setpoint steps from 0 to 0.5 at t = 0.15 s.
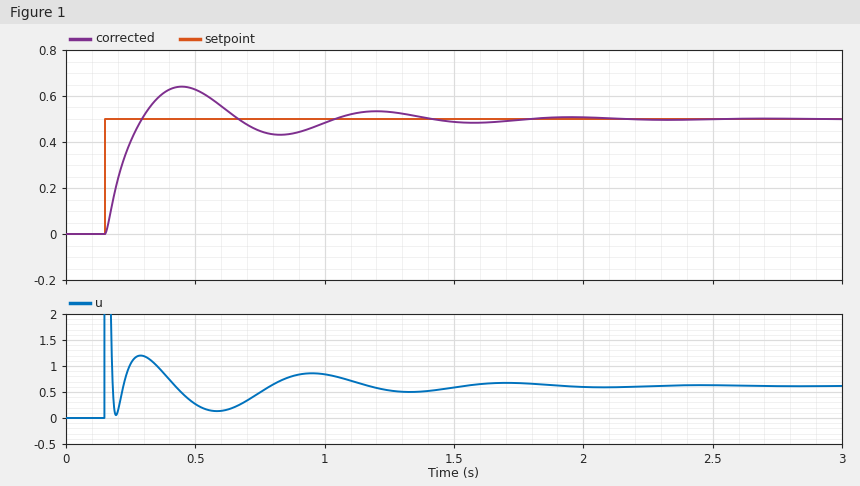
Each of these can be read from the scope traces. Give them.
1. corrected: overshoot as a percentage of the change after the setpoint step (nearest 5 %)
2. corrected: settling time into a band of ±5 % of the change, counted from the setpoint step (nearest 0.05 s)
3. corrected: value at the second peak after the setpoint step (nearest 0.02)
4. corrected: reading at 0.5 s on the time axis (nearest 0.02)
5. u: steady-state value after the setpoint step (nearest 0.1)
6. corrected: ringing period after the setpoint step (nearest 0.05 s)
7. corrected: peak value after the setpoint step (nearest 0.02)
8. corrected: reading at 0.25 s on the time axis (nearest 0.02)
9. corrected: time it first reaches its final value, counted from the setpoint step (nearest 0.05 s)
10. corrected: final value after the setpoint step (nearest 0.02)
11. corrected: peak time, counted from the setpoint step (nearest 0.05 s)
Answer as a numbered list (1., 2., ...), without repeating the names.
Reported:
1. 30 %
2. 1.15 s
3. 0.54
4. 0.62
5. 0.6
6. 0.75 s
7. 0.64
8. 0.40
9. 0.15 s
10. 0.50
11. 0.30 s
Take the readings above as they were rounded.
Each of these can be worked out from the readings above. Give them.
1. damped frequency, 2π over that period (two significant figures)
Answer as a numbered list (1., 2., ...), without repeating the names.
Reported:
1. 8.4 rad/s
